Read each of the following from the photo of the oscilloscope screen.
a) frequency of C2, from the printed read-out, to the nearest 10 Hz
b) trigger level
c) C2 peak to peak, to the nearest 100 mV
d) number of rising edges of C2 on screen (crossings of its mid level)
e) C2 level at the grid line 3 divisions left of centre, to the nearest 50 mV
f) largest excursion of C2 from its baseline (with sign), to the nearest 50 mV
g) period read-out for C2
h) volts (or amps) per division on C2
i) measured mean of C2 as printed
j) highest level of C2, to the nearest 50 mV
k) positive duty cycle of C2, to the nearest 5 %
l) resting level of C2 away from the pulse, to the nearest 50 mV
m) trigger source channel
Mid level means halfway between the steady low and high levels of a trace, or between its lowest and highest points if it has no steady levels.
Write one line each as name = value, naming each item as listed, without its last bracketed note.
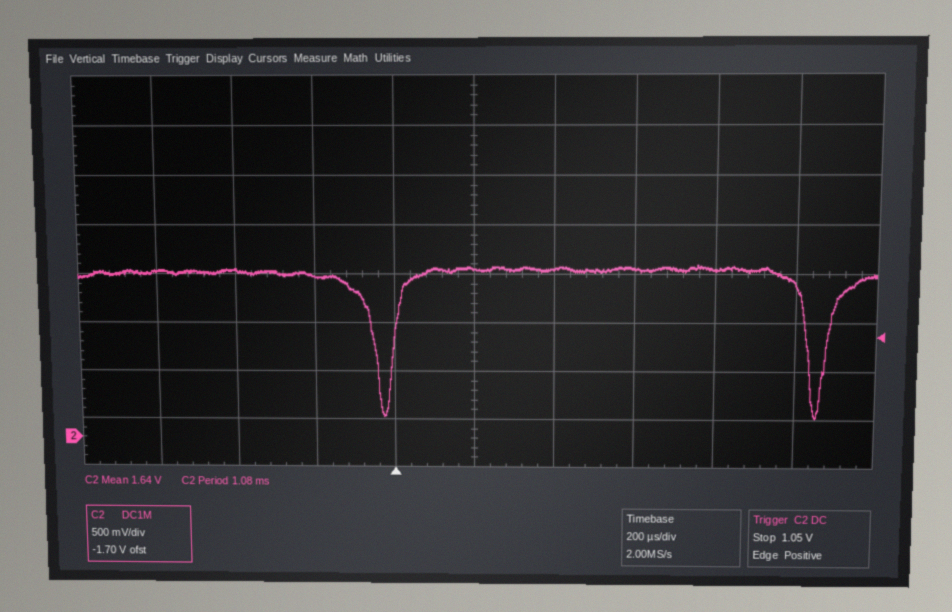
frequency of C2, from the printed read-out, to the nearest 10 Hz = 930 Hz
trigger level = 1.05 V
C2 peak to peak, to the nearest 100 mV = 1.60 V
number of rising edges of C2 on screen = 2
C2 level at the grid line 3 divisions left of centre, to the nearest 50 mV = 1.75 V
largest excursion of C2 from its baseline (with sign), to the nearest 50 mV = -1.50 V
period read-out for C2 = 1.08 ms
volts (or amps) per division on C2 = 500 mV
measured mean of C2 as printed = 1.64 V
highest level of C2, to the nearest 50 mV = 1.80 V
positive duty cycle of C2, to the nearest 5 % = 95 %
resting level of C2 away from the pulse, to the nearest 50 mV = 1.75 V
trigger source channel = C2
